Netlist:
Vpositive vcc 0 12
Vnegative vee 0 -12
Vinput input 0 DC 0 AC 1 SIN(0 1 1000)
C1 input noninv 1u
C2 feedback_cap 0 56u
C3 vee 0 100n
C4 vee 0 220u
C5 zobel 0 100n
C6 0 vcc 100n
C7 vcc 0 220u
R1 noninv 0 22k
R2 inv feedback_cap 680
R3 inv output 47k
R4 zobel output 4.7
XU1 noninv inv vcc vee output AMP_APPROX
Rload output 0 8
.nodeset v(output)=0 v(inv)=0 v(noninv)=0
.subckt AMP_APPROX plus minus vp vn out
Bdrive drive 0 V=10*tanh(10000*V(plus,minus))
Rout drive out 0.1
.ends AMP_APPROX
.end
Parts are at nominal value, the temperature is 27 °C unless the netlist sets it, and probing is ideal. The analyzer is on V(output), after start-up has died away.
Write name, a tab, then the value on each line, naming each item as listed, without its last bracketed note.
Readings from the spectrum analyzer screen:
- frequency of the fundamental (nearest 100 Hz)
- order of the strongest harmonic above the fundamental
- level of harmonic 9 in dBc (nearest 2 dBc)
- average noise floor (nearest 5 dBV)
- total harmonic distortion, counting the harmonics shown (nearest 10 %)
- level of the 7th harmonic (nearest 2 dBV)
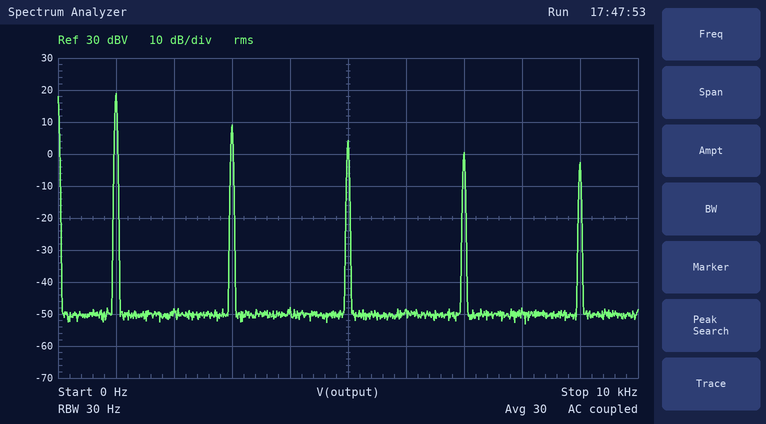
frequency of the fundamental	1.0 kHz
order of the strongest harmonic above the fundamental	3
level of harmonic 9 in dBc	-22 dBc
average noise floor	-50 dBV
total harmonic distortion, counting the harmonics shown	40 %
level of the 7th harmonic	0 dBV
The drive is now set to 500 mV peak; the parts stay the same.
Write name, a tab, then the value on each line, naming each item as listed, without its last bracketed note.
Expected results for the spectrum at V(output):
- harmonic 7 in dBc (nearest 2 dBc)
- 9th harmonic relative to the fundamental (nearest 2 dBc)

harmonic 7 in dBc	-24 dBc
9th harmonic relative to the fundamental	-32 dBc
